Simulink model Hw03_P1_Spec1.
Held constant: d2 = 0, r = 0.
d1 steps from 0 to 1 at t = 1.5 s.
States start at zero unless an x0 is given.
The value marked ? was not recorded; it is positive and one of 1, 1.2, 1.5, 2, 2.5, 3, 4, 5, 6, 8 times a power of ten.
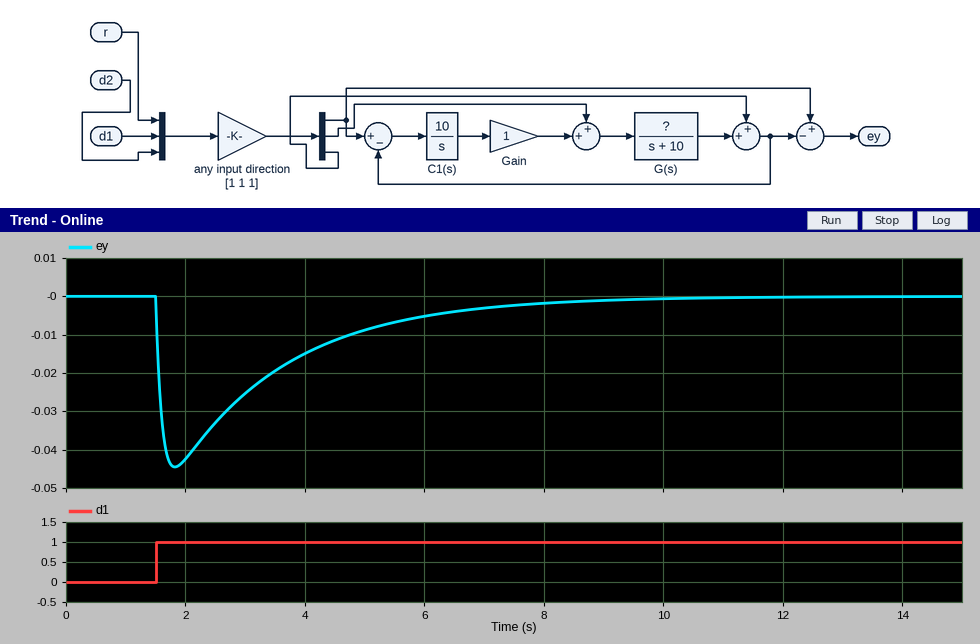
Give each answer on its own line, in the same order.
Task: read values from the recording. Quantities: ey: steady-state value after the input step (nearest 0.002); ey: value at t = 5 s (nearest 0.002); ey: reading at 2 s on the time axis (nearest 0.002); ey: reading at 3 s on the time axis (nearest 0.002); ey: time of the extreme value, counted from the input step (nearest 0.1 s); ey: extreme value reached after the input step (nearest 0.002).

0.000
-0.008
-0.042
-0.026
0.3 s
-0.044
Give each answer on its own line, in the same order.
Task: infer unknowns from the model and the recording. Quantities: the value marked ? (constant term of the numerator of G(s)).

0.5
